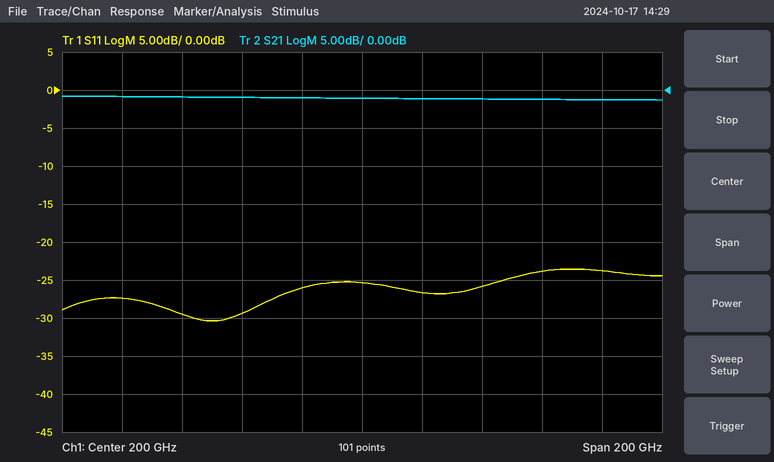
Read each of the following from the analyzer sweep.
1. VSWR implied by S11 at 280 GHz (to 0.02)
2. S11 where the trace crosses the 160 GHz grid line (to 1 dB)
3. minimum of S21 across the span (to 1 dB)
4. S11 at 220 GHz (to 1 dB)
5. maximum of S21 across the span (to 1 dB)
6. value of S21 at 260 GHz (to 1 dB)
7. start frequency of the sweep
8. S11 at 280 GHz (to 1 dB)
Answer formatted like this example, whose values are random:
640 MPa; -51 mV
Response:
1.14; -29 dB; -1 dB; -27 dB; -1 dB; -1 dB; 100 GHz; -24 dB
